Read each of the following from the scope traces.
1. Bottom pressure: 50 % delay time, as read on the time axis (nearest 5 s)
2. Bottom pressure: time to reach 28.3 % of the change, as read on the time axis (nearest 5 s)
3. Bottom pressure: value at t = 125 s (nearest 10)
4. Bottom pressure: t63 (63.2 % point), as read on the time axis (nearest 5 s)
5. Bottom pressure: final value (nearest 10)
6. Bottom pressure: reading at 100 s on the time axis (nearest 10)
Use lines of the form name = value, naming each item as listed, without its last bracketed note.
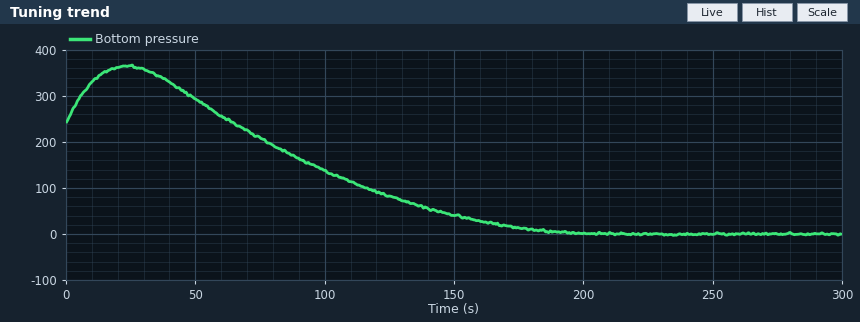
Bottom pressure: 50 % delay time, as read on the time axis = 105 s
Bottom pressure: time to reach 28.3 % of the change, as read on the time axis = 85 s
Bottom pressure: value at t = 125 s = 80
Bottom pressure: t63 (63.2 % point), as read on the time axis = 120 s
Bottom pressure: final value = 0
Bottom pressure: reading at 100 s on the time axis = 140
